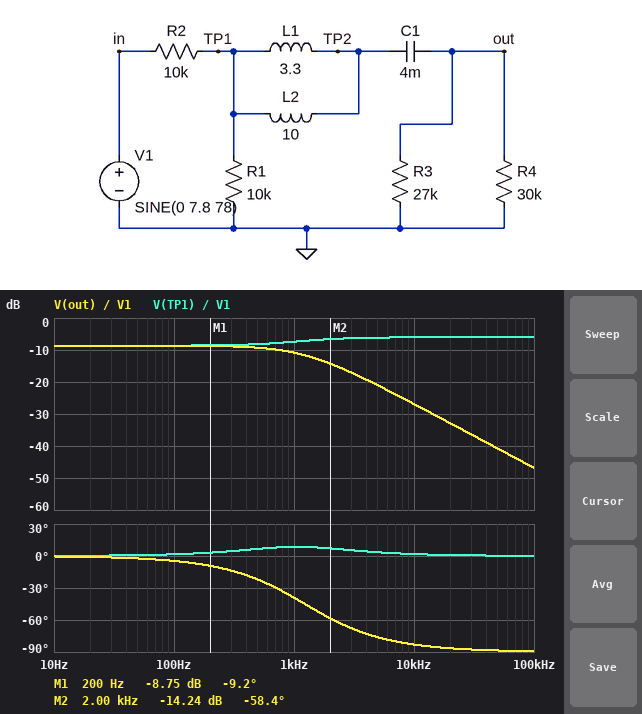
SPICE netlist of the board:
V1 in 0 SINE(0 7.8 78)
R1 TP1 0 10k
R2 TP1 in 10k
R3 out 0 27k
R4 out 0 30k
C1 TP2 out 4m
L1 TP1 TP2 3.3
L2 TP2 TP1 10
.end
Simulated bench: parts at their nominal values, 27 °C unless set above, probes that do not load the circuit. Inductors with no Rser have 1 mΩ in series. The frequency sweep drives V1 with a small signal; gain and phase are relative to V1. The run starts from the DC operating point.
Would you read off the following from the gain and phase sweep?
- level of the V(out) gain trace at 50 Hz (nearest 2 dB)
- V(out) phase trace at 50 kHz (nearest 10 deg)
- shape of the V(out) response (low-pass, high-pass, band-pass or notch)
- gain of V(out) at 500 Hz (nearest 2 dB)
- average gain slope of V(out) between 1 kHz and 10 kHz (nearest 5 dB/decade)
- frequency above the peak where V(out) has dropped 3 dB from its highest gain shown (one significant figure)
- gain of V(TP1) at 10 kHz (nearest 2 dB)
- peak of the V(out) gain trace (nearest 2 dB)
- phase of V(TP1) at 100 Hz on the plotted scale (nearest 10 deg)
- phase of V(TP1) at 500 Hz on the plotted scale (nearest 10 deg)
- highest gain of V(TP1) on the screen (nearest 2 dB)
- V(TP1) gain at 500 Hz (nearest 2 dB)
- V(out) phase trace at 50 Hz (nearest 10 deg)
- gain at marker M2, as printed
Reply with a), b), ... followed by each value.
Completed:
a) -8 dB
b) -90 deg
c) low-pass
d) -10 dB
e) -15 dB/decade
f) 1 kHz
g) -6 dB
h) -8 dB
i) 0 deg
j) 10 deg
k) -6 dB
l) -8 dB
m) 0 deg
n) -14.24 dB
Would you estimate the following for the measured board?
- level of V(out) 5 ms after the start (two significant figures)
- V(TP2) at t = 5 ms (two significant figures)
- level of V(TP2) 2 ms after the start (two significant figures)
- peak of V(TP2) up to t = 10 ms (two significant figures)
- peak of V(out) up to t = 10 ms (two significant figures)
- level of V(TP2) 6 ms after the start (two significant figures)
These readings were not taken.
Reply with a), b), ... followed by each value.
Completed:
a) 2.0 V
b) 2.0 V
c) 2.3 V
d) 2.9 V
e) 2.9 V
f) 750 mV
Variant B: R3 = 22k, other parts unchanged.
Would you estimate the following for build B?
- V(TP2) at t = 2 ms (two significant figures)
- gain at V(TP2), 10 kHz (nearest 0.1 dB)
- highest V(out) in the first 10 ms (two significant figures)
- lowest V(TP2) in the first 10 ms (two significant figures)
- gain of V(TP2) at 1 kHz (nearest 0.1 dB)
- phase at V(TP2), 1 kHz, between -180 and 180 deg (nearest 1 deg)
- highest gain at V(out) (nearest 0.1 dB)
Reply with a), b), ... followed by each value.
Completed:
a) 2.2 V
b) -27.9 dB
c) 2.8 V
d) -2.8 V
e) -11.4 dB
f) -41 deg
g) -8.9 dB
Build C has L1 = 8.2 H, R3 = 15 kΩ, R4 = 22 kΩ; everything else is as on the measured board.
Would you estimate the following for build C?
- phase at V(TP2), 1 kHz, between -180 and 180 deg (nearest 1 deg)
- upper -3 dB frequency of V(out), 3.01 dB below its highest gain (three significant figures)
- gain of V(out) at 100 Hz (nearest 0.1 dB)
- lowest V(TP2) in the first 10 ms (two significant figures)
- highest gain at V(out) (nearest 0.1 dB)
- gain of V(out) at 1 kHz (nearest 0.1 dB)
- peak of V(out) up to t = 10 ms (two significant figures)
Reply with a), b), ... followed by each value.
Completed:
a) -64 deg
b) 492 Hz
c) -10.1 dB
d) -2.5 V
e) -9.9 dB
f) -17.0 dB
g) 2.5 V
